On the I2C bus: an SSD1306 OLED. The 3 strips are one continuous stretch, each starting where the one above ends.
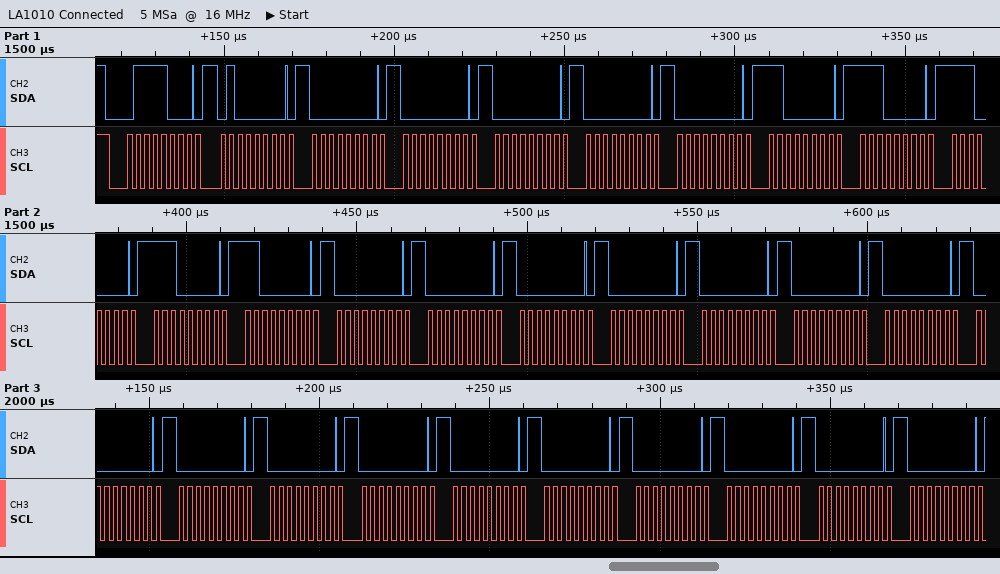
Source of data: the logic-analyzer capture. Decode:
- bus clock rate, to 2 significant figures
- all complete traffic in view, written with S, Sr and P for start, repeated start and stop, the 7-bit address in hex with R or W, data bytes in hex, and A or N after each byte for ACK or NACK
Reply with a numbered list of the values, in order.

1. 400 kHz
2. S 3CW A 40 A 00 A 00 A 00 A 00 A 00 A C0 A E0 A E0 A E0 A C0 A 00 A 00 A 00 A 00 A 00 A 00 A 00 A 00 A 00 A 00 A 00 A 00 A 00 A 00 A 00 A 00 A 00 A
